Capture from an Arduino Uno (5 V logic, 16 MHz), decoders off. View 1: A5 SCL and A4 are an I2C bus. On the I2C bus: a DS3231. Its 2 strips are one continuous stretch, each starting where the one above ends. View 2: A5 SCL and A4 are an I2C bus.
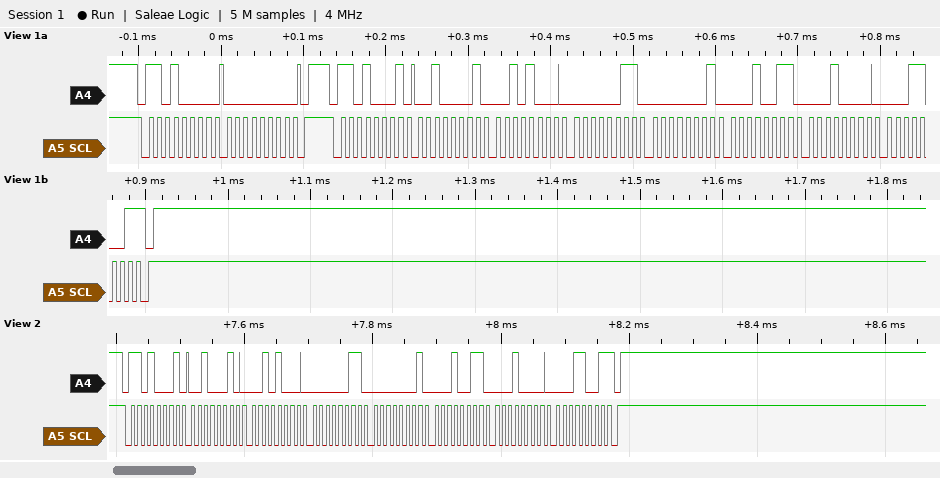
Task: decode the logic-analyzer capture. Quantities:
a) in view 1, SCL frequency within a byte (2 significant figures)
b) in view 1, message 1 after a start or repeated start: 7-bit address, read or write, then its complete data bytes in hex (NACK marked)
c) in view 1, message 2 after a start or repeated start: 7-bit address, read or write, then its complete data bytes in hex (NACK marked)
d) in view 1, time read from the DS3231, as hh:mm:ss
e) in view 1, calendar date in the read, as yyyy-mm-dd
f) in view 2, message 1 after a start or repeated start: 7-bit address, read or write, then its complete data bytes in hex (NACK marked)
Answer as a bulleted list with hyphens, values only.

- 100 kHz
- 0x68 write: 00
- 0x68 read: 21 28 03 01 13 10 19 NACK
- 03:28:21
- 2019-10-13
- 0x68 read: 22 28 03 01 13 10 19 NACK
